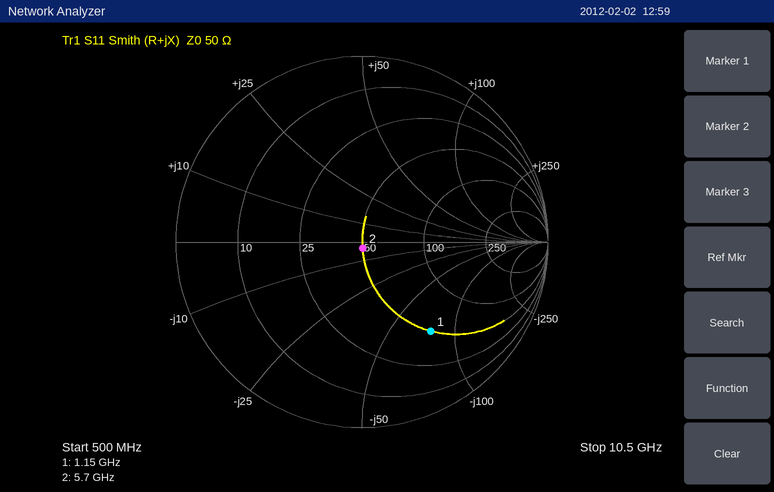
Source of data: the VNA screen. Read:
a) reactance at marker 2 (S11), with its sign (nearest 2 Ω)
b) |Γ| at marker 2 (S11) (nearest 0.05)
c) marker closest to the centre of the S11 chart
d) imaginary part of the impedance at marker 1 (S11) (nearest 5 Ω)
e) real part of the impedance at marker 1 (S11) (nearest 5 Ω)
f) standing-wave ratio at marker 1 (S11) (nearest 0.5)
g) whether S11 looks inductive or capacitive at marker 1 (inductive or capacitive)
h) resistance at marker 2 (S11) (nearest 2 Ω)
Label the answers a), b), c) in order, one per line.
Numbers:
a) -4 Ω
b) 0.05
c) marker 2
d) -75 Ω
e) 50 Ω
f) 4.0
g) capacitive
h) 50 Ω
